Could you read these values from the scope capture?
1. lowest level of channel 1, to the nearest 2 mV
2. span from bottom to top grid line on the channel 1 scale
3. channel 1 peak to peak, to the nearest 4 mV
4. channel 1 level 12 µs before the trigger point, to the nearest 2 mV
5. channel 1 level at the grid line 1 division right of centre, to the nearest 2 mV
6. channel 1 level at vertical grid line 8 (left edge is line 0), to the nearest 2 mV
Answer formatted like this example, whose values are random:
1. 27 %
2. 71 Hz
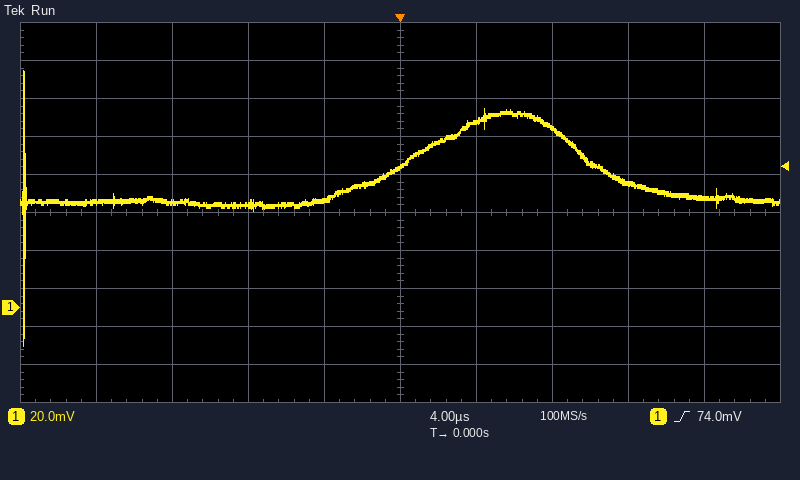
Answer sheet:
1. -20 mV
2. 200 mV
3. 144 mV
4. 56 mV
5. 98 mV
6. 66 mV
